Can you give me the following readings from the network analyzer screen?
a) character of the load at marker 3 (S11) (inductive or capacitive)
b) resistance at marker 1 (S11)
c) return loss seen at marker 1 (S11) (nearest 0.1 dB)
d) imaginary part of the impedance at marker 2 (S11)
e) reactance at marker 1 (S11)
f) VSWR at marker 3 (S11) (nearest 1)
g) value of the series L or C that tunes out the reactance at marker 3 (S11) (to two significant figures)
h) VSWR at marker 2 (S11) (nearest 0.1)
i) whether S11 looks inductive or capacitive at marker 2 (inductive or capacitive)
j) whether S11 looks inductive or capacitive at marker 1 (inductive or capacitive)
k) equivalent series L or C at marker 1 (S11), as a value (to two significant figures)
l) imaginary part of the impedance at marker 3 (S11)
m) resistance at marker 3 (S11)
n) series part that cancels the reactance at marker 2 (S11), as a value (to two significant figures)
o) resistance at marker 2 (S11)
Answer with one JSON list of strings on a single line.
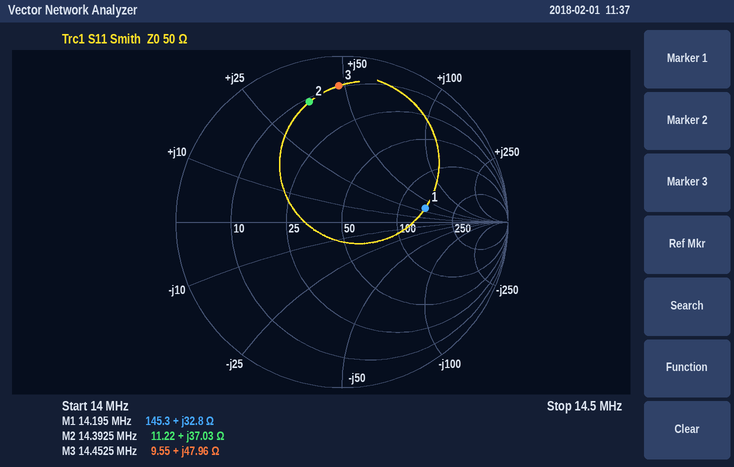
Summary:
["inductive", "145.3 Ω", "5.9 dB", "+37.03 Ω", "+32.8 Ω", "10", "230 pF", "7.0", "inductive", "inductive", "370 nH", "+47.96 Ω", "9.55 Ω", "300 pF", "11.22 Ω"]
